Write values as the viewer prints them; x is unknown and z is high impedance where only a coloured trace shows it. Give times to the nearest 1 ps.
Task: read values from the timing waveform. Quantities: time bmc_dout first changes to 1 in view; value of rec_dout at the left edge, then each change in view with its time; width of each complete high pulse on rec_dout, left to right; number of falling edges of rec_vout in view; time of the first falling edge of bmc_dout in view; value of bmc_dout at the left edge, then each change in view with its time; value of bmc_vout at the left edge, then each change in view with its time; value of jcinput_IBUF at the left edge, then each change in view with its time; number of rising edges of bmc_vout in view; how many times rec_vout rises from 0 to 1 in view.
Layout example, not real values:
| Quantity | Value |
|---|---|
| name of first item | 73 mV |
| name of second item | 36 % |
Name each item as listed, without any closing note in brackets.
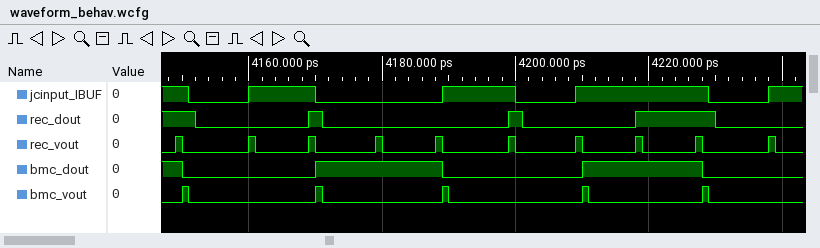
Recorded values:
| Quantity | Value |
|---|---|
| time bmc_dout first changes to 1 in view | 4170 ps |
| value of rec_dout at the left edge, then each change in view with its time | 1, 0 at 4152 ps, 1 at 4169 ps, 0 at 4171 ps, 1 at 4199 ps, 0 at 4201 ps, 1 at 4218 ps, 0 at 4230 ps |
| width of each complete high pulse on rec_dout, left to right | 2 ps, 2 ps, 12 ps |
| number of falling edges of rec_vout in view | 10 |
| time of the first falling edge of bmc_dout in view | 4150 ps |
| value of bmc_dout at the left edge, then each change in view with its time | 1, 0 at 4150 ps, 1 at 4170 ps, 0 at 4189 ps, 1 at 4210 ps, 0 at 4228 ps |
| value of bmc_vout at the left edge, then each change in view with its time | 0, 1 at 4150 ps, 0 at 4151 ps, 1 at 4170 ps, 0 at 4171 ps, 1 at 4189 ps, 0 at 4190 ps, 1 at 4210 ps, 0 at 4211 ps, 1 at 4228 ps, 0 at 4229 ps |
| value of jcinput_IBUF at the left edge, then each change in view with its time | 1, 0 at 4151 ps, 1 at 4160 ps, 0 at 4170 ps, 1 at 4189 ps, 0 at 4200 ps, 1 at 4209 ps, 0 at 4229 ps, 1 at 4238 ps |
| number of rising edges of bmc_vout in view | 5 |
| how many times rec_vout rises from 0 to 1 in view | 10 |
